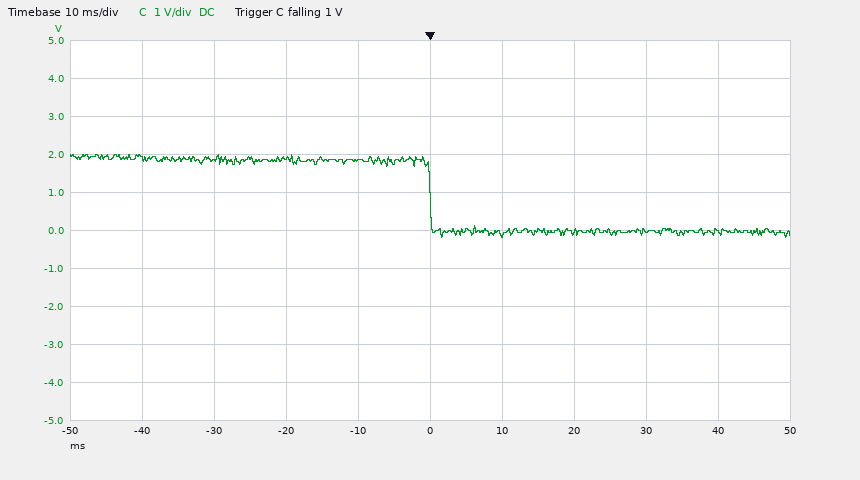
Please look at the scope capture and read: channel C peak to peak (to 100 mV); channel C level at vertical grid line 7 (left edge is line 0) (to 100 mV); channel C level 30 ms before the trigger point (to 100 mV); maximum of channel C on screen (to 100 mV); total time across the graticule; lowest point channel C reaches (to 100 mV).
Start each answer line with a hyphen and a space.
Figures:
- 2.2 V
- 0.0 V
- 1.9 V
- 2.0 V
- 100 ms
- -200 mV
